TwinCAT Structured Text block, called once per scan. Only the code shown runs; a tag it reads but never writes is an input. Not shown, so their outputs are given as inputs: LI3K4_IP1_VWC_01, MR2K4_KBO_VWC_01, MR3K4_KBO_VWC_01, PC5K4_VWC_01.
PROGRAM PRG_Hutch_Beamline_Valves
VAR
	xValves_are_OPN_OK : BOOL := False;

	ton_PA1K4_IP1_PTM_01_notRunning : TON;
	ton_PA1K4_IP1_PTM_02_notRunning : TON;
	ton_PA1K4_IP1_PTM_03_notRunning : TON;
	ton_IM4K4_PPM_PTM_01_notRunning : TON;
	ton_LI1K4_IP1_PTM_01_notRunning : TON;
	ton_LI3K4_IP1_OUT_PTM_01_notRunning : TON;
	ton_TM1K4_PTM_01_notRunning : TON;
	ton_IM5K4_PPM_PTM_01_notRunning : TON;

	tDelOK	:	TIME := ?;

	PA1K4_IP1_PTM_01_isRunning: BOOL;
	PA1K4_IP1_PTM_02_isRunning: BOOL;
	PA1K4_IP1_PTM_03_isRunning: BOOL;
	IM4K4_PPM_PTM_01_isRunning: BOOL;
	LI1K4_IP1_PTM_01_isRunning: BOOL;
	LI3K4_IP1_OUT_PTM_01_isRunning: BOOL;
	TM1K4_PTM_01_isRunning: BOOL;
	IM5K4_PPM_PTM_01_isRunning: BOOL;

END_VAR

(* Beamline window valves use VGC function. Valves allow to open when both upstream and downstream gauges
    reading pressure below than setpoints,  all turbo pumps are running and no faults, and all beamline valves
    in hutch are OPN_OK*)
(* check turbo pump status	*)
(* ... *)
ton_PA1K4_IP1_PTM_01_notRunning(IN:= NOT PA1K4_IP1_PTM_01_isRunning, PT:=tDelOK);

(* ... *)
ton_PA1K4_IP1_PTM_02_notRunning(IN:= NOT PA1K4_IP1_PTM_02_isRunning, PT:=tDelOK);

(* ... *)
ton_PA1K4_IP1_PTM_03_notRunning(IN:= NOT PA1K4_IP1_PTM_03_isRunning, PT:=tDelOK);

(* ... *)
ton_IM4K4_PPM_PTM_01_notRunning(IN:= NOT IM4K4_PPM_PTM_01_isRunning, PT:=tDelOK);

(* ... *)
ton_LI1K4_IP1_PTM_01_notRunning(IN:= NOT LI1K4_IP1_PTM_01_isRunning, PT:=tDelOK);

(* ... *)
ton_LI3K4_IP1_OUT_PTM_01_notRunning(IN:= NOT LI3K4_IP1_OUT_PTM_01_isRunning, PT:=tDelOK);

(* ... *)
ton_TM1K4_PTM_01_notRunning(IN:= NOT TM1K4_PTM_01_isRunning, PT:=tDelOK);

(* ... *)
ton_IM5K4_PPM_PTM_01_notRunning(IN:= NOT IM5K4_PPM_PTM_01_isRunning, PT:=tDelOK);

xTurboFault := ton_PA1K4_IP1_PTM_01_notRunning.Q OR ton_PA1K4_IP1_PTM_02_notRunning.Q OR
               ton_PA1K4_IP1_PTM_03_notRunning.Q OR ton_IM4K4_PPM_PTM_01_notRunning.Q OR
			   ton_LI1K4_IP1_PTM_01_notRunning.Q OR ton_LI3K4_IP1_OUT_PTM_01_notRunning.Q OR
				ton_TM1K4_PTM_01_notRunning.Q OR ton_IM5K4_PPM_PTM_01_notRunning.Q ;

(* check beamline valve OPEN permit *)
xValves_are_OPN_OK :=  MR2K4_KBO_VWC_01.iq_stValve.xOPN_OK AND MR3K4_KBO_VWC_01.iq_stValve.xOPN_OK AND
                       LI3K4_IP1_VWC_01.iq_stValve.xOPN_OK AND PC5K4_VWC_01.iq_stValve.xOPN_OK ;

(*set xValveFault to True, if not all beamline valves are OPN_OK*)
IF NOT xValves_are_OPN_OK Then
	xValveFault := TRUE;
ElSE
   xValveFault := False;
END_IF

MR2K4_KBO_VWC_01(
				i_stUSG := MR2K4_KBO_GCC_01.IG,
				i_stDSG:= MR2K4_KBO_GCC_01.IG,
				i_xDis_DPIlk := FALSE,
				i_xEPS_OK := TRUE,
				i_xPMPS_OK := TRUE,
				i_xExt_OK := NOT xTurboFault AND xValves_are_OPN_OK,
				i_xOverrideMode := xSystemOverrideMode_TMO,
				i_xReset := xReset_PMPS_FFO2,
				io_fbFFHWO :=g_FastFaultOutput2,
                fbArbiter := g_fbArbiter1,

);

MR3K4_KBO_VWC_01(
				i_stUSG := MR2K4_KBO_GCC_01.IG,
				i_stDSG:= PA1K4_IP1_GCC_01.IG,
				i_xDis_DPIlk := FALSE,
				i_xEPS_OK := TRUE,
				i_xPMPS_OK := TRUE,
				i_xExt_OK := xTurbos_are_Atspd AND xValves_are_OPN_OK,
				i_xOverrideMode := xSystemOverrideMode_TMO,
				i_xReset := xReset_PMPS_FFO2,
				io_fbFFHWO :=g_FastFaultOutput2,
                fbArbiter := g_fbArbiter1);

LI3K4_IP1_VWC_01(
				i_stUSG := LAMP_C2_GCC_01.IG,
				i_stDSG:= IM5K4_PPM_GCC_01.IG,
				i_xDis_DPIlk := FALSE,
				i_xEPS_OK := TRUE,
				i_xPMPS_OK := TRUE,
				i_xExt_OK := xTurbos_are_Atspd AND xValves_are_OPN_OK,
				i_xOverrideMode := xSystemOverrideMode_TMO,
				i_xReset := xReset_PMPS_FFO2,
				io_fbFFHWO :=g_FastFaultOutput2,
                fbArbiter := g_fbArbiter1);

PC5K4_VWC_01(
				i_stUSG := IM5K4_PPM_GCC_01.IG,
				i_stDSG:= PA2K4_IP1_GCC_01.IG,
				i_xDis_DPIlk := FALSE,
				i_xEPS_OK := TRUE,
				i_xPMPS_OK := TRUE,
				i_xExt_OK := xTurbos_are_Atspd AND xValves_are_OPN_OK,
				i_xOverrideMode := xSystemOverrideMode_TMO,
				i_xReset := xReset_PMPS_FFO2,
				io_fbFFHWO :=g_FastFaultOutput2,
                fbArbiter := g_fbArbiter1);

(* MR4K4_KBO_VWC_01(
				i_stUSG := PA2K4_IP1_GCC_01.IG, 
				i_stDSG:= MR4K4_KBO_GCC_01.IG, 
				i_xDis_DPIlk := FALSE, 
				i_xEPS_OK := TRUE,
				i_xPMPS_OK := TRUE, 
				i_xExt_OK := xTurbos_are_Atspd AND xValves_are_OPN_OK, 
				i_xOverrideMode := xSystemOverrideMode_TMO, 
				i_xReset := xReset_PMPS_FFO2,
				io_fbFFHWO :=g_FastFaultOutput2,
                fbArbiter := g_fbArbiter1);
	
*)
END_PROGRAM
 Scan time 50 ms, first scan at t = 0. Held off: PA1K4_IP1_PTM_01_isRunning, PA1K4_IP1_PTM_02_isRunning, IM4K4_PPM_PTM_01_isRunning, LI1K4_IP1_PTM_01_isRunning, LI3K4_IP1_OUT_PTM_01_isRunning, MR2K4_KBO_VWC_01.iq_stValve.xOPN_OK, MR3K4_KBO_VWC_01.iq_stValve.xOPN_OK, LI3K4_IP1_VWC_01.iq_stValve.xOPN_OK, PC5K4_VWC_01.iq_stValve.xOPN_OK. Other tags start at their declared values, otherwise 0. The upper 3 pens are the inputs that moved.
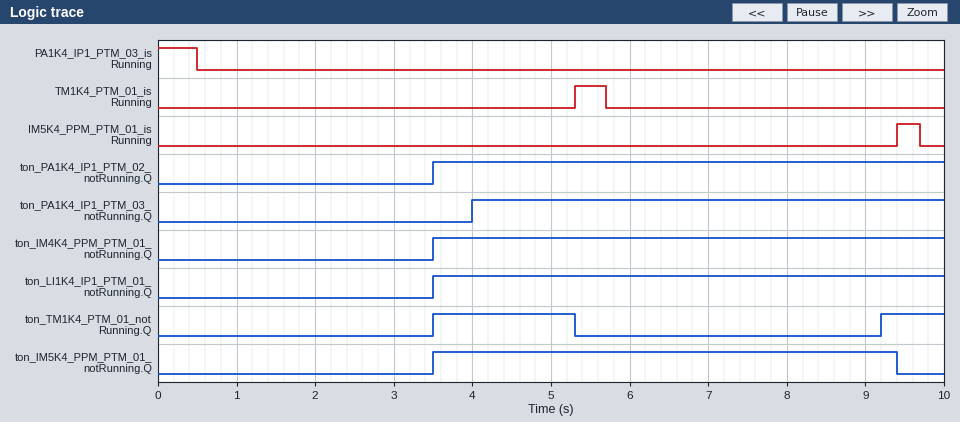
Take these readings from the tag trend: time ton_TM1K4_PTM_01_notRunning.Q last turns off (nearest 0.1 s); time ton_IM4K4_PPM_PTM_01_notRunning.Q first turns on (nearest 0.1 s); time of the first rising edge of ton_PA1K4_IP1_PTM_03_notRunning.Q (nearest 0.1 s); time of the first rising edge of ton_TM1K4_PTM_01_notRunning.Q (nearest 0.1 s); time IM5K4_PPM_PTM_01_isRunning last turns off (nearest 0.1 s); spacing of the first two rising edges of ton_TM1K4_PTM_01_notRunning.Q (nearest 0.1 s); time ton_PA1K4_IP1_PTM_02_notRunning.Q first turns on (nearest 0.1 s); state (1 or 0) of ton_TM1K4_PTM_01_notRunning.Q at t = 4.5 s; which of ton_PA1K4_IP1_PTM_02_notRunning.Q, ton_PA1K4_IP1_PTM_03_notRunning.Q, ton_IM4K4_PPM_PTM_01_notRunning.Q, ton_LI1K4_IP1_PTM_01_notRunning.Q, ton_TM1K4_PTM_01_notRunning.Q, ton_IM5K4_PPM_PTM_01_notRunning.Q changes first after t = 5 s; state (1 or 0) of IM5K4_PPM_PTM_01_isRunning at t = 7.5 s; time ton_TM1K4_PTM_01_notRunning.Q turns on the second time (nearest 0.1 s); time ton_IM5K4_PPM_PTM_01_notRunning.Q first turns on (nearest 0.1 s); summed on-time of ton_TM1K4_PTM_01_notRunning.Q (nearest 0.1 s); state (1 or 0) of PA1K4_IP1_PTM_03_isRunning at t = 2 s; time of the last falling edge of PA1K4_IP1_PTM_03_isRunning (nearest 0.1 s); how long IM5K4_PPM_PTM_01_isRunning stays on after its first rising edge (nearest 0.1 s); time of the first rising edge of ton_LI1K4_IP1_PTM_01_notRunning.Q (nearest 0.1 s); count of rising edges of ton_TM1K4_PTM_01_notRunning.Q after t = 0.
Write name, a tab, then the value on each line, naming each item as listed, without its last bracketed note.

time ton_TM1K4_PTM_01_notRunning.Q last turns off	5.3 s
time ton_IM4K4_PPM_PTM_01_notRunning.Q first turns on	3.5 s
time of the first rising edge of ton_PA1K4_IP1_PTM_03_notRunning.Q	4.0 s
time of the first rising edge of ton_TM1K4_PTM_01_notRunning.Q	3.5 s
time IM5K4_PPM_PTM_01_isRunning last turns off	9.7 s
spacing of the first two rising edges of ton_TM1K4_PTM_01_notRunning.Q	5.7 s
time ton_PA1K4_IP1_PTM_02_notRunning.Q first turns on	3.5 s
state (1 or 0) of ton_TM1K4_PTM_01_notRunning.Q at t = 4.5 s	1
which of ton_PA1K4_IP1_PTM_02_notRunning.Q, ton_PA1K4_IP1_PTM_03_notRunning.Q, ton_IM4K4_PPM_PTM_01_notRunning.Q, ton_LI1K4_IP1_PTM_01_notRunning.Q, ton_TM1K4_PTM_01_notRunning.Q, ton_IM5K4_PPM_PTM_01_notRunning.Q changes first after t = 5 s	ton_TM1K4_PTM_01_notRunning.Q
state (1 or 0) of IM5K4_PPM_PTM_01_isRunning at t = 7.5 s	0
time ton_TM1K4_PTM_01_notRunning.Q turns on the second time	9.2 s
time ton_IM5K4_PPM_PTM_01_notRunning.Q first turns on	3.5 s
summed on-time of ton_TM1K4_PTM_01_notRunning.Q	2.6 s
state (1 or 0) of PA1K4_IP1_PTM_03_isRunning at t = 2 s	0
time of the last falling edge of PA1K4_IP1_PTM_03_isRunning	0.5 s
how long IM5K4_PPM_PTM_01_isRunning stays on after its first rising edge	0.3 s
time of the first rising edge of ton_LI1K4_IP1_PTM_01_notRunning.Q	3.5 s
count of rising edges of ton_TM1K4_PTM_01_notRunning.Q after t = 0	2
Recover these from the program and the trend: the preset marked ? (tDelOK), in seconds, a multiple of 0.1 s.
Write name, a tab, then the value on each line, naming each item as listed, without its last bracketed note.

the preset marked ? (tDelOK), in seconds, a multiple of 0.1 s	3.5 s
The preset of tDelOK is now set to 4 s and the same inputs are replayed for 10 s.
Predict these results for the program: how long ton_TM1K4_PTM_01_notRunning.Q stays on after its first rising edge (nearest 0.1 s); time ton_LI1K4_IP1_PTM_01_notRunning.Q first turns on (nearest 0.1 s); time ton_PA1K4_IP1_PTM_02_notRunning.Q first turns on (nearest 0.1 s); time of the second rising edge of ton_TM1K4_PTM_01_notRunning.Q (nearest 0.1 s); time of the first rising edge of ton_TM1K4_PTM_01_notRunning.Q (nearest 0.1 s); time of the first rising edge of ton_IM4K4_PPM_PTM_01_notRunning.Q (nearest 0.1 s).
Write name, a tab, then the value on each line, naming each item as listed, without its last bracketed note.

how long ton_TM1K4_PTM_01_notRunning.Q stays on after its first rising edge	1.3 s
time ton_LI1K4_IP1_PTM_01_notRunning.Q first turns on	4.0 s
time ton_PA1K4_IP1_PTM_02_notRunning.Q first turns on	4.0 s
time of the second rising edge of ton_TM1K4_PTM_01_notRunning.Q	9.7 s
time of the first rising edge of ton_TM1K4_PTM_01_notRunning.Q	4.0 s
time of the first rising edge of ton_IM4K4_PPM_PTM_01_notRunning.Q	4.0 s
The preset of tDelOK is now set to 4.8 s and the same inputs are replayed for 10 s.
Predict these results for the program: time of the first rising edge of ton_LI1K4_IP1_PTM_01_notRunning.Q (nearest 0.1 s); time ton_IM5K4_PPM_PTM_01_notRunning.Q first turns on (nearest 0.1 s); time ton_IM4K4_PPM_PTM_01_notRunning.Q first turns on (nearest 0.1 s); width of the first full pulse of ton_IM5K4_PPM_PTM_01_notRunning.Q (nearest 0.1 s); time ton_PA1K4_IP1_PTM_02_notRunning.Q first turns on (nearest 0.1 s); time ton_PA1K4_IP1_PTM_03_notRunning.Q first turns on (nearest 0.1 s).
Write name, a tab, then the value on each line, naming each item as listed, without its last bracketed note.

time of the first rising edge of ton_LI1K4_IP1_PTM_01_notRunning.Q	4.8 s
time ton_IM5K4_PPM_PTM_01_notRunning.Q first turns on	4.8 s
time ton_IM4K4_PPM_PTM_01_notRunning.Q first turns on	4.8 s
width of the first full pulse of ton_IM5K4_PPM_PTM_01_notRunning.Q	4.6 s
time ton_PA1K4_IP1_PTM_02_notRunning.Q first turns on	4.8 s
time ton_PA1K4_IP1_PTM_03_notRunning.Q first turns on	5.3 s
